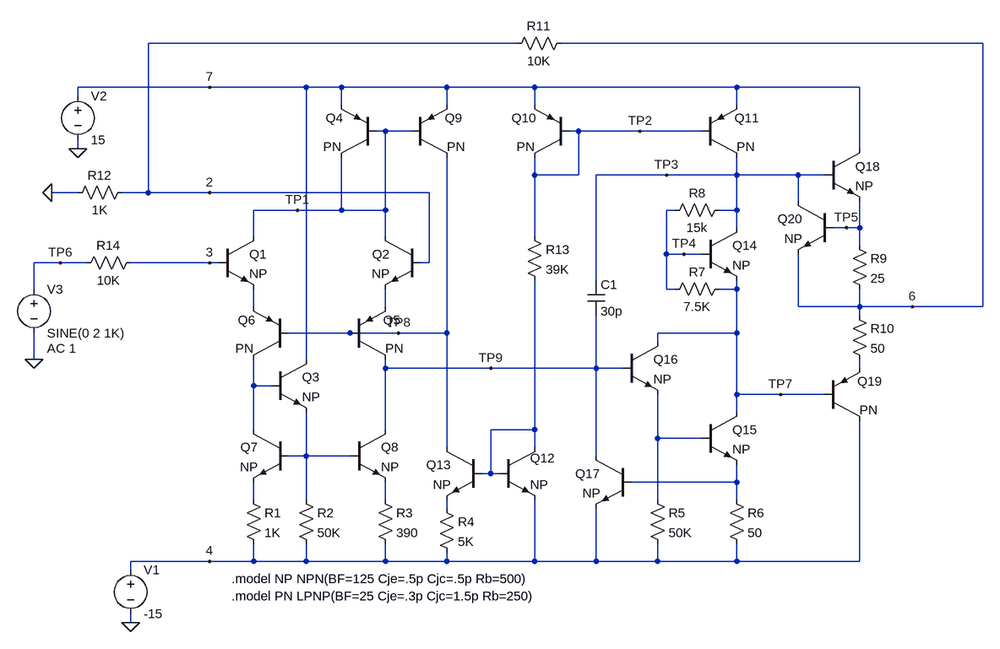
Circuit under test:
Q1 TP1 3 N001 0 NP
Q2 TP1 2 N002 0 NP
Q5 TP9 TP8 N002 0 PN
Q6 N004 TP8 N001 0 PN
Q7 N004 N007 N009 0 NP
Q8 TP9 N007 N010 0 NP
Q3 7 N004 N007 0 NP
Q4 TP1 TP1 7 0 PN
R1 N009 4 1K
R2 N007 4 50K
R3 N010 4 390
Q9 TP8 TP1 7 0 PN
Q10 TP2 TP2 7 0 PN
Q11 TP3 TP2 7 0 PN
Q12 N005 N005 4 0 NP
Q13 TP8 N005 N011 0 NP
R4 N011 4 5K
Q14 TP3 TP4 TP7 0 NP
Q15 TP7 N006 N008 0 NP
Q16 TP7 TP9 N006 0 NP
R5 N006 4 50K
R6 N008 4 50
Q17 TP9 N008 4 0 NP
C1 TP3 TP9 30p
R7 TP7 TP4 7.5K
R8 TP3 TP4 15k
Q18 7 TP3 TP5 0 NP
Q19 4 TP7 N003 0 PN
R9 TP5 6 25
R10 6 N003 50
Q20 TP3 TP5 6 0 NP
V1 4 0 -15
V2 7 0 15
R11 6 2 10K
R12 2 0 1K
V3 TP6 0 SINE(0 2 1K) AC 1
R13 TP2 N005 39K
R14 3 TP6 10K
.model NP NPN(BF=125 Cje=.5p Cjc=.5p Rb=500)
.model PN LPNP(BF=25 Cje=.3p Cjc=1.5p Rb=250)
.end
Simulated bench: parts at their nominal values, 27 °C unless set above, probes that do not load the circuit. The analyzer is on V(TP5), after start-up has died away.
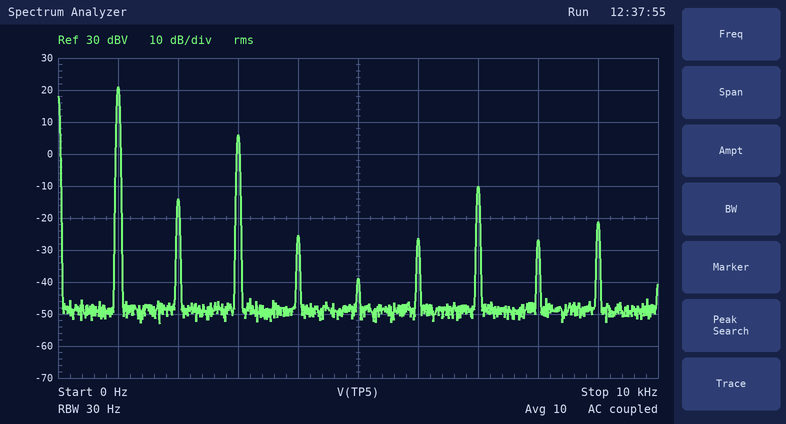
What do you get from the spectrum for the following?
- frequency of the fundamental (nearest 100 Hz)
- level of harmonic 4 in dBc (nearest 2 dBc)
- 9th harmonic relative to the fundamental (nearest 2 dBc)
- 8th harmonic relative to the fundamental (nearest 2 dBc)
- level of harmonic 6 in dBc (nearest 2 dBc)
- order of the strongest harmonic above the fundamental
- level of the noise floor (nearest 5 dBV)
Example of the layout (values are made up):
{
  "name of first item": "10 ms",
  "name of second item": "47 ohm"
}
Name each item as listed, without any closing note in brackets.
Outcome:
{
  "frequency of the fundamental": "1.0 kHz",
  "level of harmonic 4 in dBc": "-46 dBc",
  "9th harmonic relative to the fundamental": "-42 dBc",
  "8th harmonic relative to the fundamental": "-48 dBc",
  "level of harmonic 6 in dBc": "-48 dBc",
  "order of the strongest harmonic above the fundamental": "3",
  "level of the noise floor": "-50 dBV"
}
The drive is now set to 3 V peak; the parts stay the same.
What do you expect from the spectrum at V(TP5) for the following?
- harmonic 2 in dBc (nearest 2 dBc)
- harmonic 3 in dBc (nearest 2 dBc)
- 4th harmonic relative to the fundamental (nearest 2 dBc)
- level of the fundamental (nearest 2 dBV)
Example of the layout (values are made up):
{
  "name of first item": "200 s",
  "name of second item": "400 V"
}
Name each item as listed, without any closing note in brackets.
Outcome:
{
  "harmonic 2 in dBc": "-38 dBc",
  "harmonic 3 in dBc": "-12 dBc",
  "4th harmonic relative to the fundamental": "-42 dBc",
  "level of the fundamental": "22 dBV"
}
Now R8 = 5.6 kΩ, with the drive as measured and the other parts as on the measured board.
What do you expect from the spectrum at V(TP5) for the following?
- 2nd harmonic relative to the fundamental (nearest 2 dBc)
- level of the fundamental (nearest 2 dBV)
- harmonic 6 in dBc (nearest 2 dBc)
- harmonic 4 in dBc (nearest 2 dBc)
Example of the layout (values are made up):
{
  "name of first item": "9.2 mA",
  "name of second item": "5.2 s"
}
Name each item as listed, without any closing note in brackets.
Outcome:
{
  "2nd harmonic relative to the fundamental": "-38 dBc",
  "level of the fundamental": "22 dBV",
  "harmonic 6 in dBc": "-50 dBc",
  "harmonic 4 in dBc": "-50 dBc"
}
